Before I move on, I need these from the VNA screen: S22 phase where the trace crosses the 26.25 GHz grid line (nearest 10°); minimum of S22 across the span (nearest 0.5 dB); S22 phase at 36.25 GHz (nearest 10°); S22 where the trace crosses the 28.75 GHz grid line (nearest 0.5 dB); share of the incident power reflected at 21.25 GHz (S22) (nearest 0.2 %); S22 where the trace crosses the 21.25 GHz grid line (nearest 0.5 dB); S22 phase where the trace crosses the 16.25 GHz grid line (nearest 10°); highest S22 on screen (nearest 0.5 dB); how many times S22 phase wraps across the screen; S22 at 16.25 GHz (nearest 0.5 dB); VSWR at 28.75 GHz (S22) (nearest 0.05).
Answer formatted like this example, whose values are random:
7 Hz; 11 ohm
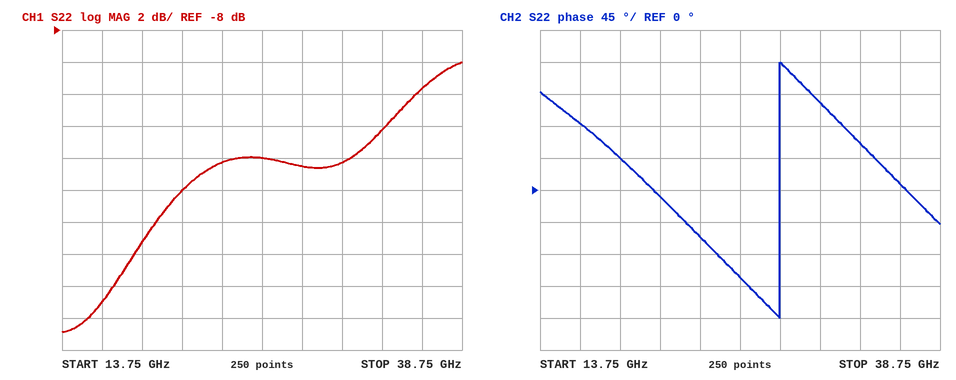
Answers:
-120°; -27.0 dB; 10°; -16.5 dB; 1.6 %; -18.0 dB; 90°; -10.0 dB; 1; -25.0 dB; 1.35
